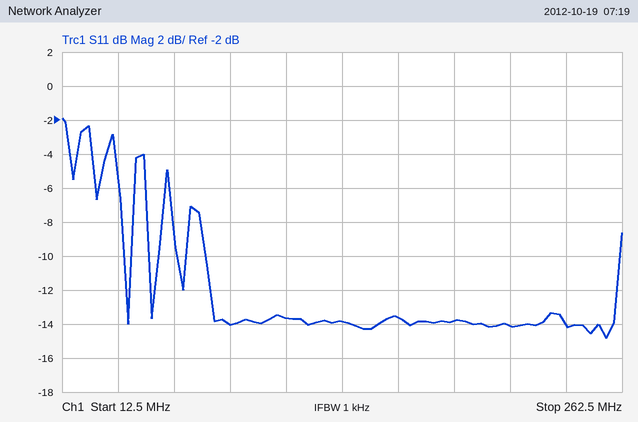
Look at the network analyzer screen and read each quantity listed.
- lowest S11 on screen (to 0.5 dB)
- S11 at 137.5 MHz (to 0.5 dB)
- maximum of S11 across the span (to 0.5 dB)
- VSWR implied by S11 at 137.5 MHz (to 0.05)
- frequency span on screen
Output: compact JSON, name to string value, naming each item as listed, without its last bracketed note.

{"lowest S11 on screen": "-15.0 dB", "S11 at 137.5 MHz": "-14.0 dB", "maximum of S11 across the span": "-2.0 dB", "VSWR implied by S11 at 137.5 MHz": "1.50", "frequency span on screen": "250 MHz"}
